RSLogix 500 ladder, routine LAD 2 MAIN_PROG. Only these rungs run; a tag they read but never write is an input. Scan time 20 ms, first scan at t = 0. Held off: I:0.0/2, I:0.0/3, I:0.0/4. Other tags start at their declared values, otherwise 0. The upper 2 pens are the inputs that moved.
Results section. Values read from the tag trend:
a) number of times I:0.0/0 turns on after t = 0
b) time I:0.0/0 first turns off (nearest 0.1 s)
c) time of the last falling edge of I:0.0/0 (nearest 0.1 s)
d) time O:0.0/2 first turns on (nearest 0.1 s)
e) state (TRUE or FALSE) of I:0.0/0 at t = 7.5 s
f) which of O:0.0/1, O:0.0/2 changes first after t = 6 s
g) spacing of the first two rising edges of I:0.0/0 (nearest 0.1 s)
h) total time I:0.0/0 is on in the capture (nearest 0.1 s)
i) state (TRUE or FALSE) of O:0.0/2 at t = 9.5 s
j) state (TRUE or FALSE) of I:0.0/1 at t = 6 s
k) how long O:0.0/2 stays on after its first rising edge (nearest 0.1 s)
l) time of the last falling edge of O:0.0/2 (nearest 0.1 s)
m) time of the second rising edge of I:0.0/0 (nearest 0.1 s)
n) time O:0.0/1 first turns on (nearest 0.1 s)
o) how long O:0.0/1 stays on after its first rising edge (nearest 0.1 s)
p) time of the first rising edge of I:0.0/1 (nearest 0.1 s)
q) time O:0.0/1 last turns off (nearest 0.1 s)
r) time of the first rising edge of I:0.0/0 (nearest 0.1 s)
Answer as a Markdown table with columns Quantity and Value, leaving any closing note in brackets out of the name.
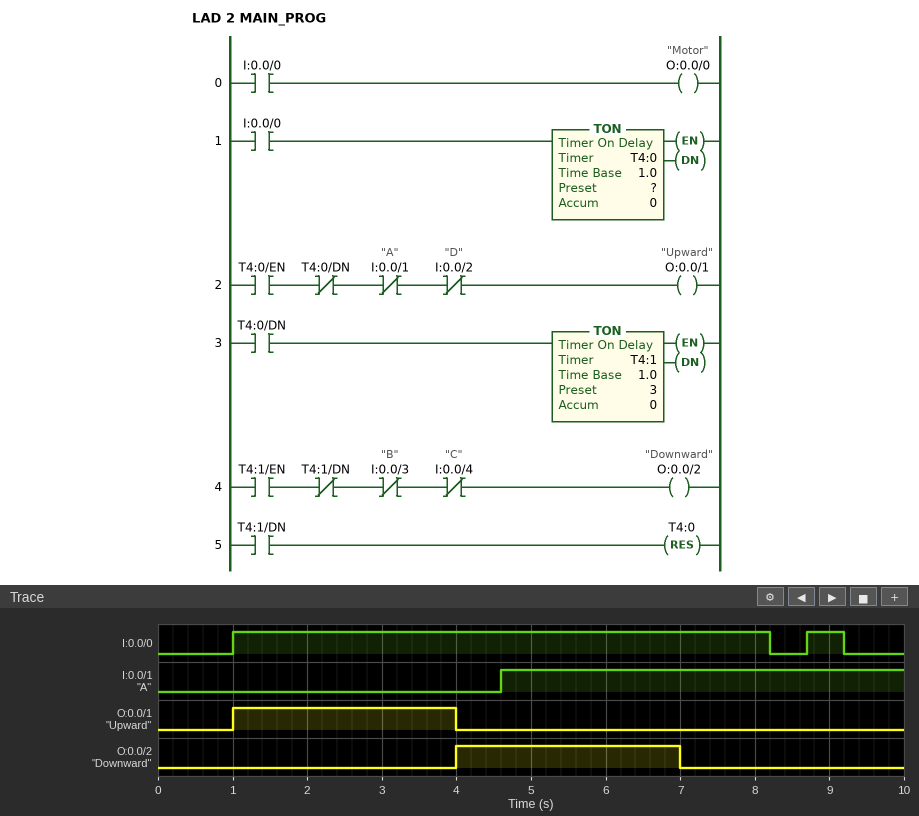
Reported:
| Quantity | Value |
|---|---|
| number of times I:0.0/0 turns on after t = 0 | 2 |
| time I:0.0/0 first turns off | 8.2 s |
| time of the last falling edge of I:0.0/0 | 9.2 s |
| time O:0.0/2 first turns on | 4.0 s |
| state (TRUE or FALSE) of I:0.0/0 at t = 7.5 s | TRUE |
| which of O:0.0/1, O:0.0/2 changes first after t = 6 s | O:0.0/2 |
| spacing of the first two rising edges of I:0.0/0 | 7.7 s |
| total time I:0.0/0 is on in the capture | 7.7 s |
| state (TRUE or FALSE) of O:0.0/2 at t = 9.5 s | FALSE |
| state (TRUE or FALSE) of I:0.0/1 at t = 6 s | TRUE |
| how long O:0.0/2 stays on after its first rising edge | 3.0 s |
| time of the last falling edge of O:0.0/2 | 7.0 s |
| time of the second rising edge of I:0.0/0 | 8.7 s |
| time O:0.0/1 first turns on | 1.0 s |
| how long O:0.0/1 stays on after its first rising edge | 3.0 s |
| time of the first rising edge of I:0.0/1 | 4.6 s |
| time O:0.0/1 last turns off | 4.0 s |
| time of the first rising edge of I:0.0/0 | 1.0 s |
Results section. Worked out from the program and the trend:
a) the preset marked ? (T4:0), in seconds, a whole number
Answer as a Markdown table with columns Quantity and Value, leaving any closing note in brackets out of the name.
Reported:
| Quantity | Value |
|---|---|
| the preset marked ? (T4:0), in seconds, a whole number | 3 s |
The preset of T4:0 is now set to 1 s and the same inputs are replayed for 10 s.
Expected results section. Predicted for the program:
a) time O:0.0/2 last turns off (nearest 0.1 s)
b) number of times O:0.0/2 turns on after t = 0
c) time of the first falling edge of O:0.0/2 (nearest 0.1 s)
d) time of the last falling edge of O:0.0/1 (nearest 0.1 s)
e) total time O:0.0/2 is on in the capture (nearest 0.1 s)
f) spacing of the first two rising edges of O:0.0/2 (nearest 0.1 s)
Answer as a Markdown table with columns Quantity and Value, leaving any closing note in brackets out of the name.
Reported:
| Quantity | Value |
|---|---|
| time O:0.0/2 last turns off | 8.2 s |
| number of times O:0.0/2 turns on after t = 0 | 2 |
| time of the first falling edge of O:0.0/2 | 5.0 s |
| time of the last falling edge of O:0.0/1 | 2.0 s |
| total time O:0.0/2 is on in the capture | 5.2 s |
| spacing of the first two rising edges of O:0.0/2 | 4.0 s |
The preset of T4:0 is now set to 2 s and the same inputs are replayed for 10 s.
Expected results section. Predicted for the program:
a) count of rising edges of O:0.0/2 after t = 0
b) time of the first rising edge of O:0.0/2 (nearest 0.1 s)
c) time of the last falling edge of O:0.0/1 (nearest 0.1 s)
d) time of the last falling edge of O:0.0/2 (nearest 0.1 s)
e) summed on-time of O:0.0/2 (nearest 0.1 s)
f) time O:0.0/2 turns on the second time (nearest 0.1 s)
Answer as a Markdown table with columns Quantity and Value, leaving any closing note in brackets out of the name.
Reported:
| Quantity | Value |
|---|---|
| count of rising edges of O:0.0/2 after t = 0 | 2 |
| time of the first rising edge of O:0.0/2 | 3.0 s |
| time of the last falling edge of O:0.0/1 | 3.0 s |
| time of the last falling edge of O:0.0/2 | 8.2 s |
| summed on-time of O:0.0/2 | 3.2 s |
| time O:0.0/2 turns on the second time | 8.0 s |
